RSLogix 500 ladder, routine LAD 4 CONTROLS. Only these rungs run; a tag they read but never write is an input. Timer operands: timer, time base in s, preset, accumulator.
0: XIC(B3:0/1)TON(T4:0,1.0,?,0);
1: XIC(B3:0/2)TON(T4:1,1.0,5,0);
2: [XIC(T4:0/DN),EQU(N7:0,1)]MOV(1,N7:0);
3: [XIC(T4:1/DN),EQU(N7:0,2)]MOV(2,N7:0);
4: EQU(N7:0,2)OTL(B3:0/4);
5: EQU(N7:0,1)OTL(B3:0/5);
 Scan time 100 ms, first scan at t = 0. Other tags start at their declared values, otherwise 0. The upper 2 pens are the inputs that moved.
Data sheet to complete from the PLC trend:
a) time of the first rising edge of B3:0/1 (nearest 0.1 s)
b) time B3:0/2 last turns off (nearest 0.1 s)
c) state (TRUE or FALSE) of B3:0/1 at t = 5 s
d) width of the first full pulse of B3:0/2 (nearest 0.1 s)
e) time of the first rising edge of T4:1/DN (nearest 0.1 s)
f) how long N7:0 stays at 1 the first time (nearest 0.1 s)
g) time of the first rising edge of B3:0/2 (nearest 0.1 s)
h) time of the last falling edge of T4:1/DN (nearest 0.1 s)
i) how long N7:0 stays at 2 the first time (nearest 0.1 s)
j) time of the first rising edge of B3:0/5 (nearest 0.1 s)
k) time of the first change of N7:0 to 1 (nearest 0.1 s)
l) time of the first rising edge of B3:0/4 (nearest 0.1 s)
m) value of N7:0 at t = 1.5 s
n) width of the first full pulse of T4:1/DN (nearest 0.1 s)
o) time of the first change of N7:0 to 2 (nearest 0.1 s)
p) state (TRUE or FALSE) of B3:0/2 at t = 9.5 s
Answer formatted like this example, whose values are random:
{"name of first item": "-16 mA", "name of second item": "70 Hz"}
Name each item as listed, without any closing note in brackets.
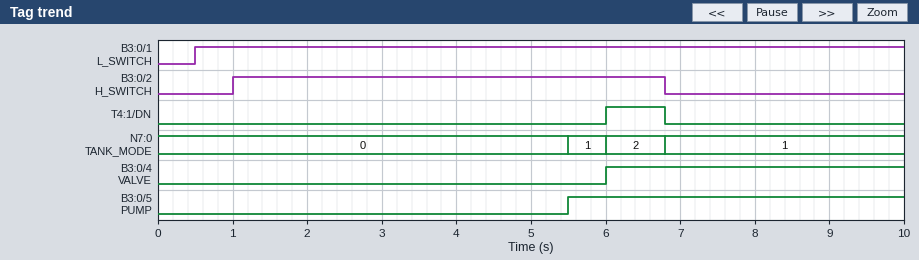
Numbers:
{"time of the first rising edge of B3:0/1": "0.5 s", "time B3:0/2 last turns off": "6.8 s", "state (TRUE or FALSE) of B3:0/1 at t = 5 s": "TRUE", "width of the first full pulse of B3:0/2": "5.8 s", "time of the first rising edge of T4:1/DN": "6.0 s", "how long N7:0 stays at 1 the first time": "0.5 s", "time of the first rising edge of B3:0/2": "1.0 s", "time of the last falling edge of T4:1/DN": "6.8 s", "how long N7:0 stays at 2 the first time": "0.8 s", "time of the first rising edge of B3:0/5": "5.5 s", "time of the first change of N7:0 to 1": "5.5 s", "time of the first rising edge of B3:0/4": "6.0 s", "value of N7:0 at t = 1.5 s": "0", "width of the first full pulse of T4:1/DN": "0.8 s", "time of the first change of N7:0 to 2": "6.0 s", "state (TRUE or FALSE) of B3:0/2 at t = 9.5 s": "FALSE"}
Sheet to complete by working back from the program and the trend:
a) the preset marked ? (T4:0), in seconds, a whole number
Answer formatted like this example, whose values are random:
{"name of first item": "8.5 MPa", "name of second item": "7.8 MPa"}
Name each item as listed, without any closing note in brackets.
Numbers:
{"the preset marked ? (T4:0), in seconds, a whole number": "5 s"}
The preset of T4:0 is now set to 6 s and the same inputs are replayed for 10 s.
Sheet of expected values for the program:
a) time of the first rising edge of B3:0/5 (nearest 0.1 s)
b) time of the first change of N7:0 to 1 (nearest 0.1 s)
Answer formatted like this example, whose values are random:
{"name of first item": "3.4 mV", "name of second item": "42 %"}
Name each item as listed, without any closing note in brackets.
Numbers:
{"time of the first rising edge of B3:0/5": "6.8 s", "time of the first change of N7:0 to 1": "6.8 s"}
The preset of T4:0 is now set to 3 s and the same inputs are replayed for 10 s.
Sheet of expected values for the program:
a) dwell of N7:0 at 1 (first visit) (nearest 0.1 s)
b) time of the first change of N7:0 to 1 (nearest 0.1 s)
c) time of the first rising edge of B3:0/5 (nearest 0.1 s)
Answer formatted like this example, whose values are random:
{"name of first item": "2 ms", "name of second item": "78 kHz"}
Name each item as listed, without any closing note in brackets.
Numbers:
{"dwell of N7:0 at 1 (first visit)": "2.5 s", "time of the first change of N7:0 to 1": "3.5 s", "time of the first rising edge of B3:0/5": "3.5 s"}
